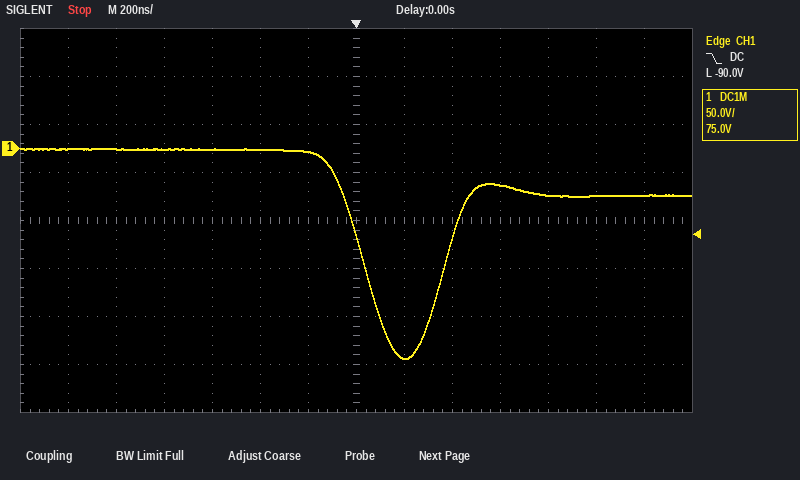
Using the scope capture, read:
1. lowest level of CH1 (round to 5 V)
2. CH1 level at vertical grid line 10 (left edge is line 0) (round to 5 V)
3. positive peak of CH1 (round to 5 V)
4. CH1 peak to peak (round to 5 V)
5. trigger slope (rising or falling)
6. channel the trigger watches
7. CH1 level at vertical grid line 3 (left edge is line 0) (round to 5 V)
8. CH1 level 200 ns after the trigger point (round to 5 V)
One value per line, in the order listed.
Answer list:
-220 V
-40 V
0 V
220 V
falling
CH1
0 V
-220 V
